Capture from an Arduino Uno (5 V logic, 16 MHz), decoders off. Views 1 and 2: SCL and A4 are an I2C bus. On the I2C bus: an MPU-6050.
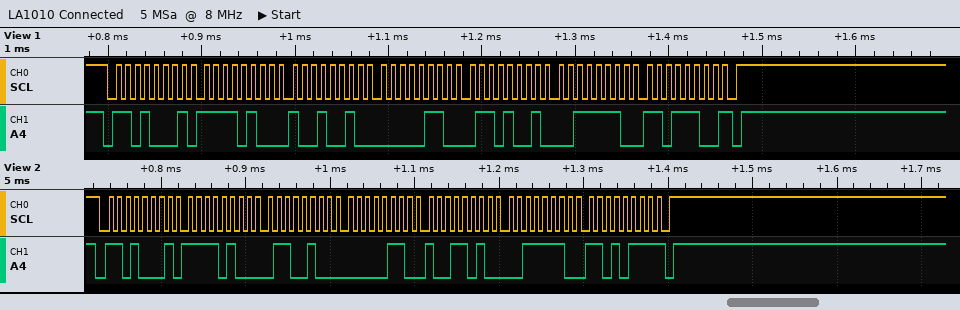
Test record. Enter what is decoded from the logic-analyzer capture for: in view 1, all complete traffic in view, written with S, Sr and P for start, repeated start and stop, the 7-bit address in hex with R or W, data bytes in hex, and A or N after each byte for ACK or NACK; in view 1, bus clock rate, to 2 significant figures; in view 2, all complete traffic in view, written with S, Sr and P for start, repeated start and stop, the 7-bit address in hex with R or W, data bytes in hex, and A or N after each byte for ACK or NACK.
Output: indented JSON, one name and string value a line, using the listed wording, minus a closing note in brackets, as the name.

{
  "in view 1, all complete traffic in view, written with S, Sr and P for start, repeated start and stop, the 7-bit address in hex with R or W, data bytes in hex, and A or N after each byte for ACK or NACK": "S 68R A F4 A 92 A 06 A 69 A 3E A DC N P",
  "in view 1, bus clock rate, to 2 significant figures": "100 kHz",
  "in view 2, all complete traffic in view, written with S, Sr and P for start, repeated start and stop, the 7-bit address in hex with R or W, data bytes in hex, and A or N after each byte for ACK or NACK": "S 68R A F4 A 64 A 06 A 9A A 3E A D7 N P"
}
